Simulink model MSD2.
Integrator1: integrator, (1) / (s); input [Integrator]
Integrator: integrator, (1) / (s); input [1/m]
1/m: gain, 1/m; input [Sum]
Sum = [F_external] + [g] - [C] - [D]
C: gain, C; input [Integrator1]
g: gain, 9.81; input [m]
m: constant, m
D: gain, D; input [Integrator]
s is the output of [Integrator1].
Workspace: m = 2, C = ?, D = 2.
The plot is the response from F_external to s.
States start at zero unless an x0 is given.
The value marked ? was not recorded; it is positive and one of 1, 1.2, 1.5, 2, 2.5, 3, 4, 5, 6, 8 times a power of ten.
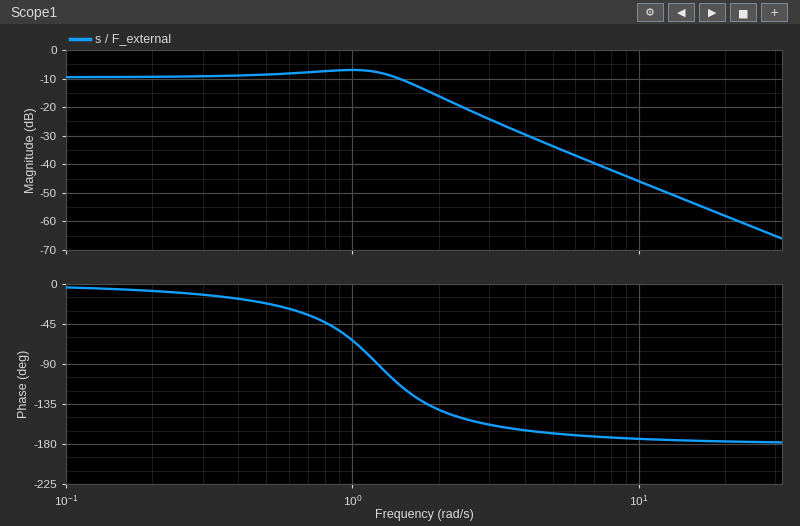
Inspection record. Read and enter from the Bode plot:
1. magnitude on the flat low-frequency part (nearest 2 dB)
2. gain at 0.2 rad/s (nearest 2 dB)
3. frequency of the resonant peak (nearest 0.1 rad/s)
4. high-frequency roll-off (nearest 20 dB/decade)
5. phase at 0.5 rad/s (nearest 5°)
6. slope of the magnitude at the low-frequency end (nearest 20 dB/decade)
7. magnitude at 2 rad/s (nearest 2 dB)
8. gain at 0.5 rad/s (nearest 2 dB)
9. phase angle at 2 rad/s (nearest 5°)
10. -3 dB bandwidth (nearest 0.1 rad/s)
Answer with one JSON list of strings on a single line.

["-10 dB", "-10 dB", "1.0 rad/s", "-40 dB/decade", "-20°", "0 dB/decade", "-16 dB", "-8 dB", "-140°", "1.7 rad/s"]
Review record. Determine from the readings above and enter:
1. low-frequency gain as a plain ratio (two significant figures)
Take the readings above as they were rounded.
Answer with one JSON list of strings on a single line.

["0.32"]
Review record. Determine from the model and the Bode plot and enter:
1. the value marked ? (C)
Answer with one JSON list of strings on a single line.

["3"]
